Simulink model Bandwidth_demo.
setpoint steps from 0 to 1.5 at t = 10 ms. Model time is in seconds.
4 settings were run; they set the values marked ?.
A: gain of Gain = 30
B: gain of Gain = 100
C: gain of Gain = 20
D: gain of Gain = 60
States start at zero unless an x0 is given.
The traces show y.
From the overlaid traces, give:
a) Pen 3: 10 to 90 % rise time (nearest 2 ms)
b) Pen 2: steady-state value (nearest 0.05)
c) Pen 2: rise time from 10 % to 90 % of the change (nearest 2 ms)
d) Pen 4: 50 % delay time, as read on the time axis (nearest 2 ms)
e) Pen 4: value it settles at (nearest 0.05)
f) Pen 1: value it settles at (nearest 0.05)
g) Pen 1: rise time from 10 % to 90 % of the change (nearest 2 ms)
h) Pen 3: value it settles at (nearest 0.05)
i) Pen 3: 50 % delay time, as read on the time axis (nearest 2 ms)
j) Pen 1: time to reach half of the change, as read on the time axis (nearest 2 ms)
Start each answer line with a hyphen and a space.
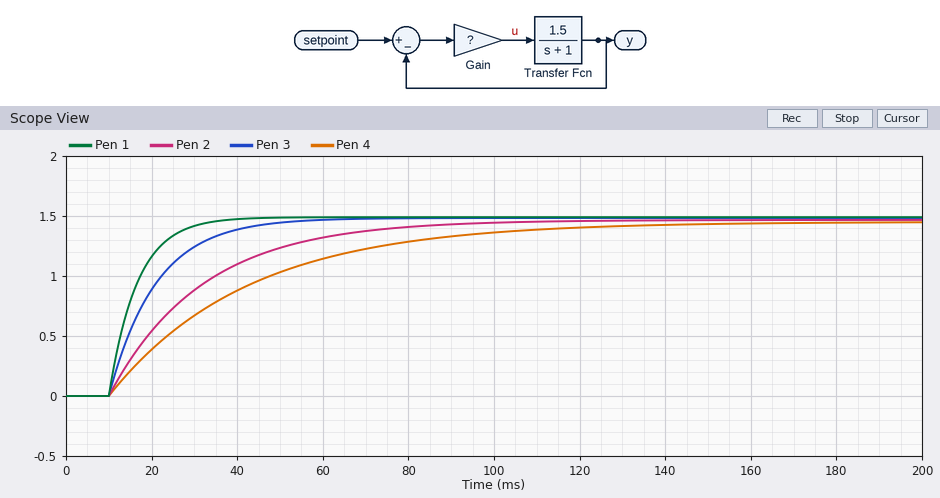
- 24 ms
- 1.45
- 48 ms
- 32 ms
- 1.45
- 1.50
- 14 ms
- 1.50
- 18 ms
- 14 ms
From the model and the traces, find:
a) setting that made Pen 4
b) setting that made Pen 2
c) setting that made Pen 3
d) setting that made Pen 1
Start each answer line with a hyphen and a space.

- C
- A
- D
- B
